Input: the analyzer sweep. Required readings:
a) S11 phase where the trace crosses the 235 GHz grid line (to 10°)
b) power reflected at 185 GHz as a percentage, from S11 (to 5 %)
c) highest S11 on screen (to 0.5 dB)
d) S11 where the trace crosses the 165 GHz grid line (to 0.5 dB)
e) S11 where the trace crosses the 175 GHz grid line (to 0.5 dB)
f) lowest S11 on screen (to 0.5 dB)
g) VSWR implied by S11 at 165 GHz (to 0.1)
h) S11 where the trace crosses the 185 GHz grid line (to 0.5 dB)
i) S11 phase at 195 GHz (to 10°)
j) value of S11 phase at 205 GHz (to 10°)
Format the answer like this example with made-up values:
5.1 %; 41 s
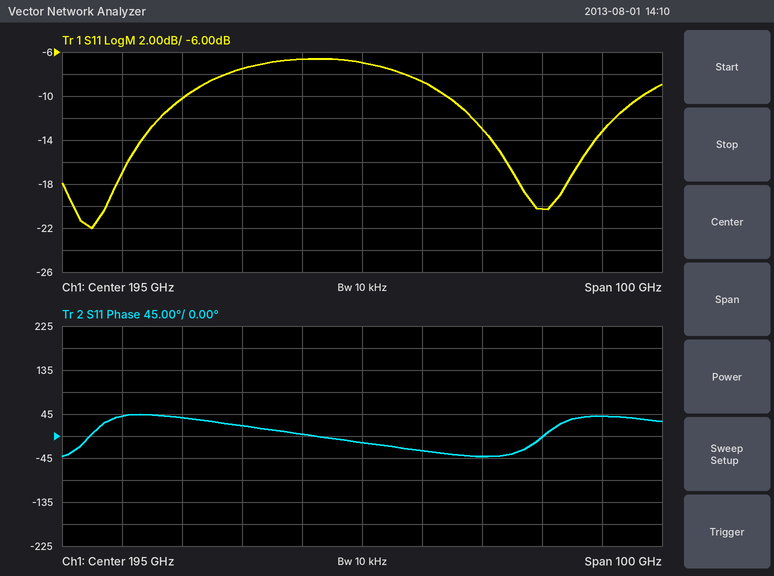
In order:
40°; 20 %; -6.5 dB; -10.0 dB; -7.5 dB; -22.0 dB; 1.9; -6.5 dB; -10°; -30°
